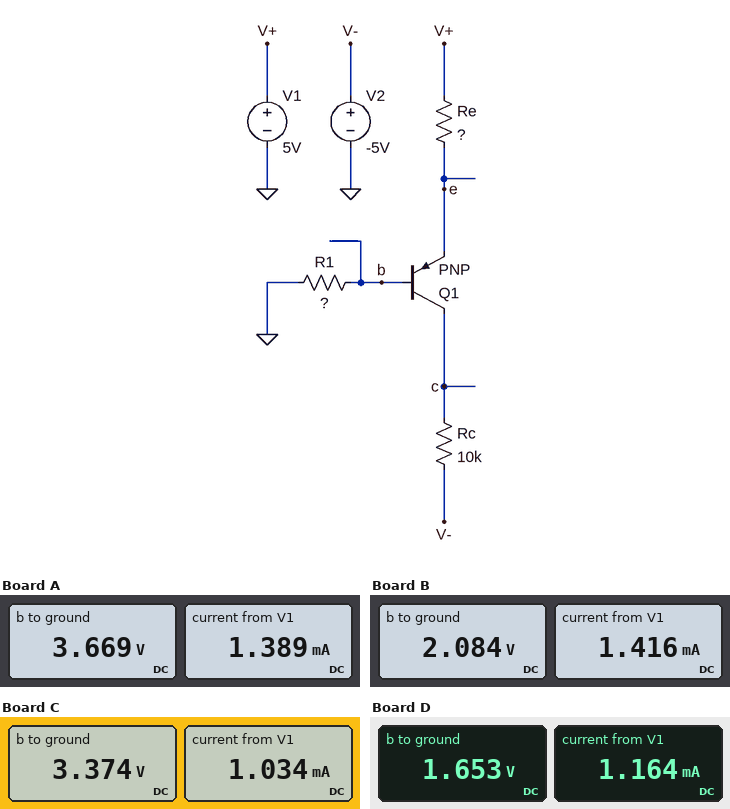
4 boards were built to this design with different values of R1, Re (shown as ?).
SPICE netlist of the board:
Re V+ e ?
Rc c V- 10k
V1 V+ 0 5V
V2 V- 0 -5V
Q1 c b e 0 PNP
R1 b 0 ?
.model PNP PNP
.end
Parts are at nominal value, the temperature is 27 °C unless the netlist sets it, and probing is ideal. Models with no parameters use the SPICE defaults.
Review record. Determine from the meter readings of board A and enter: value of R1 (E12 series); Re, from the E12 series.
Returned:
8.2 kΩ
390 Ω
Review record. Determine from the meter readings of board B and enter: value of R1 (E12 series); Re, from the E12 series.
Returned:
3.3 kΩ
1.5 kΩ
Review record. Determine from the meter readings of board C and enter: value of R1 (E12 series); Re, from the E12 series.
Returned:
27 kΩ
820 Ω
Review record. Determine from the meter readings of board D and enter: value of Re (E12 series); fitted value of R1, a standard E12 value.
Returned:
2.2 kΩ
3.9 kΩ
